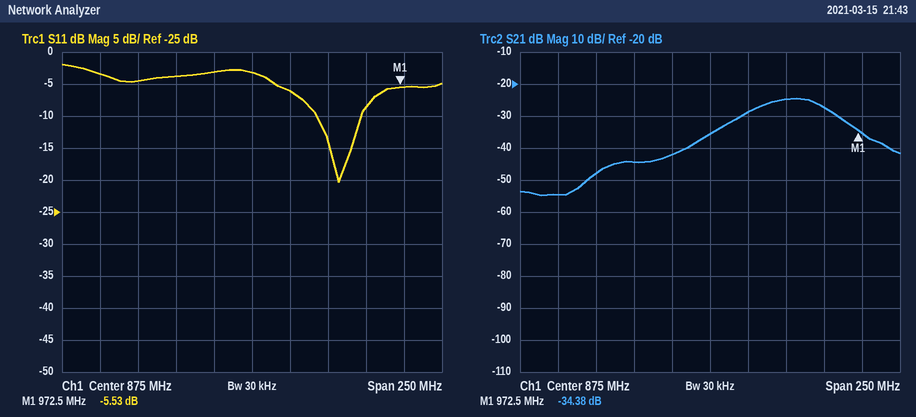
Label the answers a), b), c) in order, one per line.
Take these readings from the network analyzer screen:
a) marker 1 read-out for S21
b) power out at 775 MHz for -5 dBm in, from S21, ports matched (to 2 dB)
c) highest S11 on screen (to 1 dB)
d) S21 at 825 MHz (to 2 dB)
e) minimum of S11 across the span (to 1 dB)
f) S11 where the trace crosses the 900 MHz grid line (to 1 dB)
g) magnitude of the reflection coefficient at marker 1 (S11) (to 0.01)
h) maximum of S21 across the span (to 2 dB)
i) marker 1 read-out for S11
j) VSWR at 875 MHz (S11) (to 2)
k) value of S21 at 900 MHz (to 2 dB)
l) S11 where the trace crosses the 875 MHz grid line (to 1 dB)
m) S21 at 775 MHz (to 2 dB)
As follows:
a) -34.38 dB
b) -60 dBm
c) -2 dB
d) -44 dB
e) -20 dB
f) -6 dB
g) 0.53
h) -24 dB
i) -5.53 dB
j) 6
k) -28 dB
l) -3 dB
m) -54 dB
